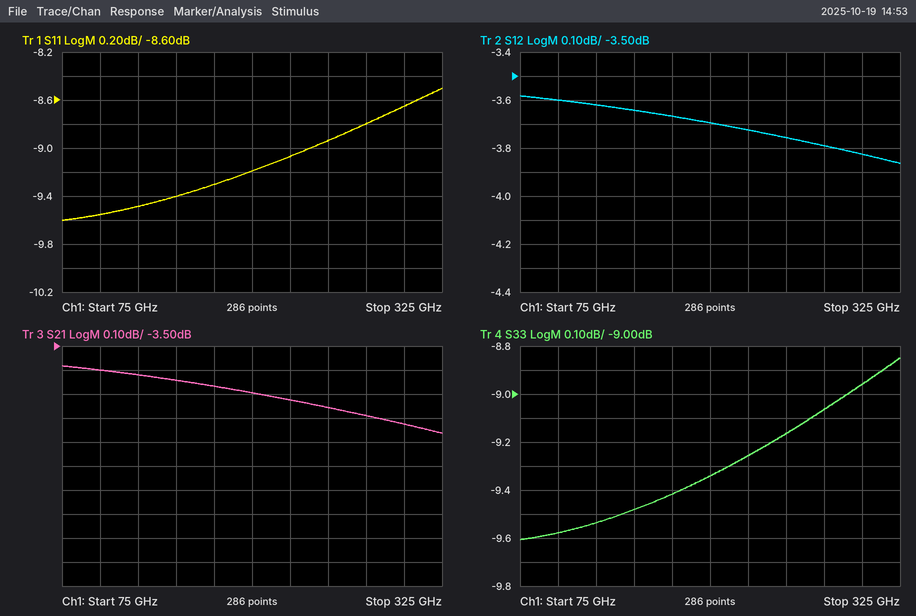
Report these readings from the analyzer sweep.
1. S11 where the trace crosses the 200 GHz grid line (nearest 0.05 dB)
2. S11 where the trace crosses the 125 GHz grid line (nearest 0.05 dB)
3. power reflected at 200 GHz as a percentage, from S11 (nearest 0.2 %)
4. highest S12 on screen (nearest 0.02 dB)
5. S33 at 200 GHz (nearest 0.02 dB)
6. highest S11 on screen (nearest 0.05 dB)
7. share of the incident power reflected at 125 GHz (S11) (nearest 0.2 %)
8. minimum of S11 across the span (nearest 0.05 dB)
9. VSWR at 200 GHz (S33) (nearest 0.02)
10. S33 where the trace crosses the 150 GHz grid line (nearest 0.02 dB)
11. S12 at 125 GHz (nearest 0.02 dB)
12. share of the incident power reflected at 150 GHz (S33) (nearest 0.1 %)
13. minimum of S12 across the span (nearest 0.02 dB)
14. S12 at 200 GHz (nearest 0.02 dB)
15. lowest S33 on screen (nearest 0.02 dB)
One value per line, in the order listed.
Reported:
-9.20 dB
-9.50 dB
12.0 %
-3.58 dB
-9.34 dB
-8.50 dB
11.2 %
-9.60 dB
2.04
-9.48 dB
-3.62 dB
11.3 %
-3.86 dB
-3.70 dB
-9.60 dB
